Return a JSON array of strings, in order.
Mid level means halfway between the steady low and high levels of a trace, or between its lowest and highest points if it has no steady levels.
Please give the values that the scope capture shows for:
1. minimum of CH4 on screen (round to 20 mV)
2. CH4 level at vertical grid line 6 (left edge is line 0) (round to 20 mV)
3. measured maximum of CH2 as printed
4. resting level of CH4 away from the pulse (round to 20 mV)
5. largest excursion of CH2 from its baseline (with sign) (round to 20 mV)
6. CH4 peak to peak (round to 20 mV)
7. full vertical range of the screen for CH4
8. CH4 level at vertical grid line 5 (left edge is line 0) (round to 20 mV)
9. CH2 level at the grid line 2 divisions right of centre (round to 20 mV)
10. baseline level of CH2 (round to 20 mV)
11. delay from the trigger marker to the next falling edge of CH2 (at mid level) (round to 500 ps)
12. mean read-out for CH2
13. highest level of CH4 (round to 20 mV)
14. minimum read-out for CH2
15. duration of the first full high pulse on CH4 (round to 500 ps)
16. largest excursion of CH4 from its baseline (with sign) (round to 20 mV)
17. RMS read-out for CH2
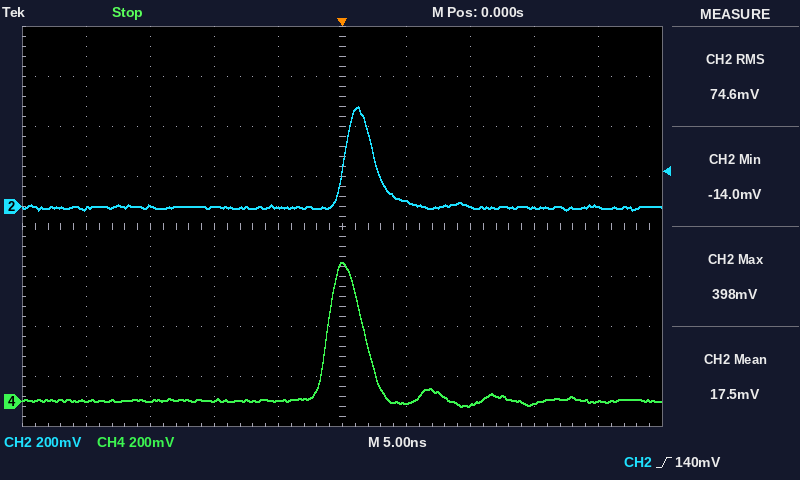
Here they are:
["-20 mV", "0 mV", "398 mV", "0 mV", "+400 mV", "580 mV", "1.6 V", "540 mV", "0 mV", "0 mV", "2.5 ns", "17.5 mV", "560 mV", "-14.0 mV", "3.0 ns", "+560 mV", "74.6 mV"]
